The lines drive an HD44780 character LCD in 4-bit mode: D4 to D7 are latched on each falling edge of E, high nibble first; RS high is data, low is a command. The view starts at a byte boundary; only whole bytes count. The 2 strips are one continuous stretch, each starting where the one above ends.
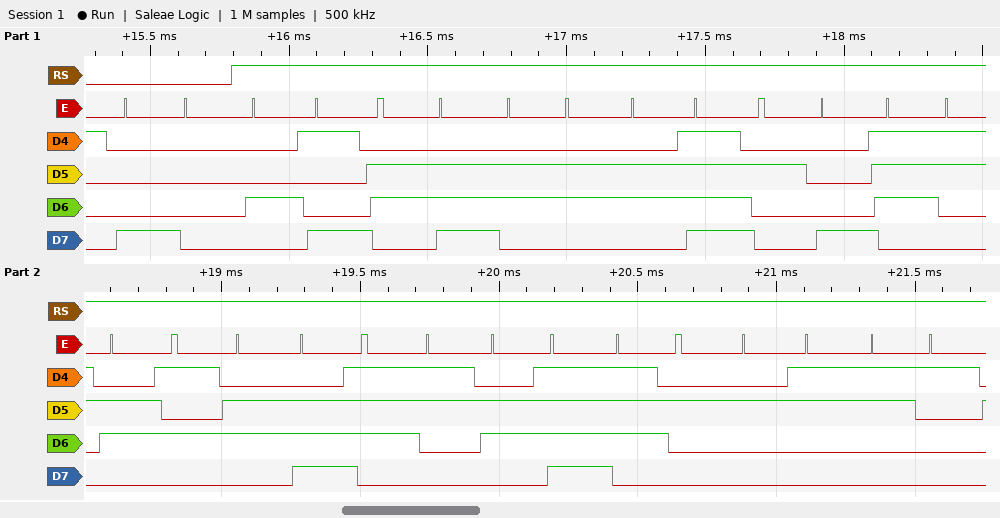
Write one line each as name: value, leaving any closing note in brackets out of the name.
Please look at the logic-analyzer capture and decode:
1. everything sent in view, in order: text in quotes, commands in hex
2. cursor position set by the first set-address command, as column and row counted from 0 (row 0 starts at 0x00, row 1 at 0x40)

everything sent in view, in order: text in quotes, commands in hex: 0x80 "Info(sensor#1"
cursor position set by the first set-address command, as column and row counted from 0: column 0, row 0
